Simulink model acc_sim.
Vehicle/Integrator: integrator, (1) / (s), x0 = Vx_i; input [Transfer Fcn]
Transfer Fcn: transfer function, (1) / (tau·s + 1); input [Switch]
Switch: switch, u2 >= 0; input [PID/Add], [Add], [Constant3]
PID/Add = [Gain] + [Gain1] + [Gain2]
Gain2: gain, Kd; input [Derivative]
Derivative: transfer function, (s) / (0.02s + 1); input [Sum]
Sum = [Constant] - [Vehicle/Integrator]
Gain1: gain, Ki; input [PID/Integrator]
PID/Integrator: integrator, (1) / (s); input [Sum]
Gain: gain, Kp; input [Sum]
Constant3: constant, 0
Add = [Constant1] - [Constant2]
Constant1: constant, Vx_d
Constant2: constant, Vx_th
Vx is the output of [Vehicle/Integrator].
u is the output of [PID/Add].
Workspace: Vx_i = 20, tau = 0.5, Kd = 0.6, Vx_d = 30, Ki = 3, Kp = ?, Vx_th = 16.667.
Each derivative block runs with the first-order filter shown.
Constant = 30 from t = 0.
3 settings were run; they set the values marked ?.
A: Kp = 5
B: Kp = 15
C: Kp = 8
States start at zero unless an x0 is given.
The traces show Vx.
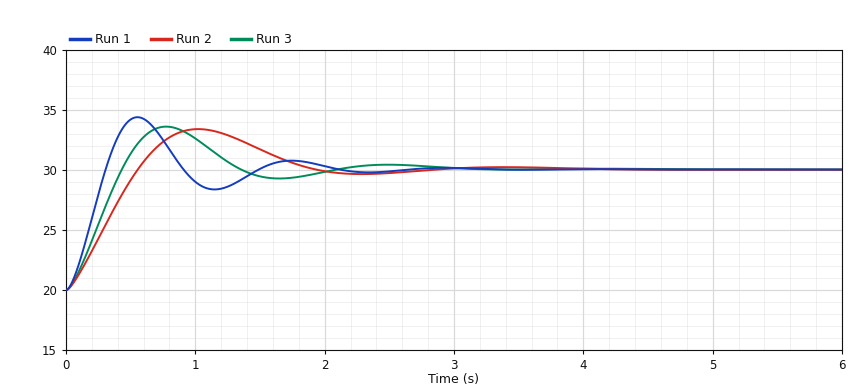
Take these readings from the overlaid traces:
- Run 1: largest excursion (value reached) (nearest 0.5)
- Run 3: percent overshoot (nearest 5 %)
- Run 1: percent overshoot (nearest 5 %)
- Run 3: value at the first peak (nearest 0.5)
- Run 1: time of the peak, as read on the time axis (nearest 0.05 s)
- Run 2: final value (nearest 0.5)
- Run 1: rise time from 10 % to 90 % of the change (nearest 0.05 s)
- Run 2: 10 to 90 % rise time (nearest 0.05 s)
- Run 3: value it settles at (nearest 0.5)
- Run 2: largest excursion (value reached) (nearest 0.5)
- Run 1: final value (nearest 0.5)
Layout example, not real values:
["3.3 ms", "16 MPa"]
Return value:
["34.5", "35 %", "45 %", "33.5", "0.55 s", "30.0", "0.20 s", "0.40 s", "30.0", "33.5", "30.0"]
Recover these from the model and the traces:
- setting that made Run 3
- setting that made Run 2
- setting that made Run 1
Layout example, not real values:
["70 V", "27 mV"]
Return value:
["C", "A", "B"]
